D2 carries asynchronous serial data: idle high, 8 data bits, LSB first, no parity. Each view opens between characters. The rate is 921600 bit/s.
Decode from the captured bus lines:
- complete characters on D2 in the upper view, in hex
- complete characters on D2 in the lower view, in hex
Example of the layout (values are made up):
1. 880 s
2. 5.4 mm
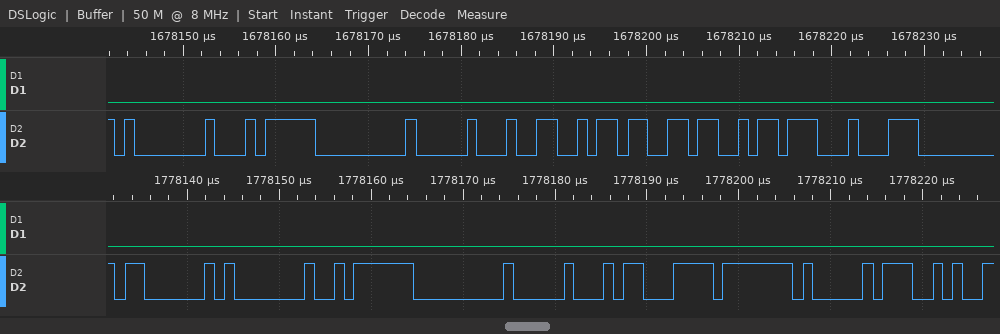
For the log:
1. 01, F4, 00, 10, A6, B3, DA, C4
2. 03, 01, FA, 00, 10, E3, 7F, D0
